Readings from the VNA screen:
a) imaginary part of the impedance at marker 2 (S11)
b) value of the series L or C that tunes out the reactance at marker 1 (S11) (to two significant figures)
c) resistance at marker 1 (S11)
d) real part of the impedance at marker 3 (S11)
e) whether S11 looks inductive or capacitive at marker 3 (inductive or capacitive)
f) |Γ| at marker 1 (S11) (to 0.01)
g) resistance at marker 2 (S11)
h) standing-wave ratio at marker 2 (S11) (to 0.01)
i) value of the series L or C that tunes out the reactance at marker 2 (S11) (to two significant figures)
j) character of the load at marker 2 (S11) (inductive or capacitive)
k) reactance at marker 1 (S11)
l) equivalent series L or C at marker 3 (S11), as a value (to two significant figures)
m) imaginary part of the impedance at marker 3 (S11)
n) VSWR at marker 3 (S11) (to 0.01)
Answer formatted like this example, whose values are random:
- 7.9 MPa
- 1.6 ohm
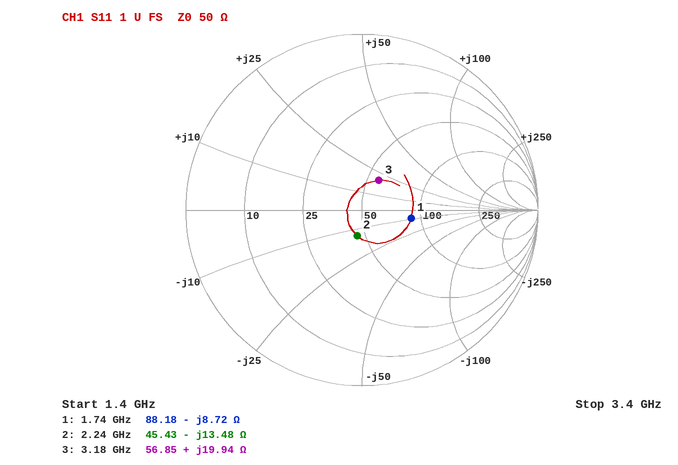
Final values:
- -13.48 Ω
- 800 pH
- 88.18 Ω
- 56.85 Ω
- inductive
- 0.28
- 45.43 Ω
- 1.35
- 960 pH
- capacitive
- -8.72 Ω
- 1.00 nH
- +19.94 Ω
- 1.48
